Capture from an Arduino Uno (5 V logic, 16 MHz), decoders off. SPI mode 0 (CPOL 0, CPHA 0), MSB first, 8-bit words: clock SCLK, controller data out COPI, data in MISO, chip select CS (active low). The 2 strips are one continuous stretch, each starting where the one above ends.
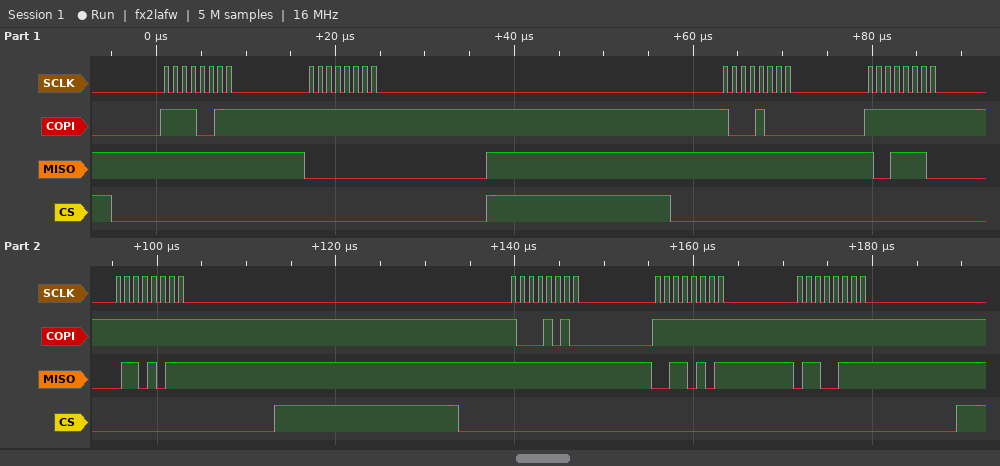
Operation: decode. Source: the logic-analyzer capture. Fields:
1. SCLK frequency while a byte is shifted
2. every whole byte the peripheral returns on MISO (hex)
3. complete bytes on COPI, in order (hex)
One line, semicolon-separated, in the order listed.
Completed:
1 MHz; FF 00 FF 9E 6B FF 35 67; F3 FF 88 FF FF 8A FF FF
